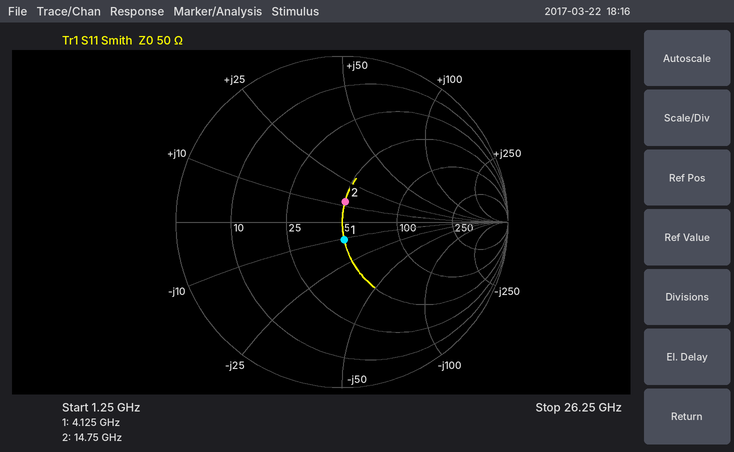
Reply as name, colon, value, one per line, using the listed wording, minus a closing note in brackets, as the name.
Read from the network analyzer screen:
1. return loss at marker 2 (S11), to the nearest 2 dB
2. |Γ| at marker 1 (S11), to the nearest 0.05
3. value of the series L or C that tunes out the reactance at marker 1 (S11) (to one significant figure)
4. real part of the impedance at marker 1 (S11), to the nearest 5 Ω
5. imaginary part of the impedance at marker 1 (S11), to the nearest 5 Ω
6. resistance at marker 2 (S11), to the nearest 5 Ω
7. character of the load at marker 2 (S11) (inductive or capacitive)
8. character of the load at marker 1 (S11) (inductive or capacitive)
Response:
return loss at marker 2 (S11), to the nearest 2 dB: 18 dB
|Γ| at marker 1 (S11), to the nearest 0.05: 0.10
value of the series L or C that tunes out the reactance at marker 1 (S11): 400 pH
real part of the impedance at marker 1 (S11), to the nearest 5 Ω: 50 Ω
imaginary part of the impedance at marker 1 (S11), to the nearest 5 Ω: -10 Ω
resistance at marker 2 (S11), to the nearest 5 Ω: 50 Ω
character of the load at marker 2 (S11): inductive
character of the load at marker 1 (S11): capacitive
